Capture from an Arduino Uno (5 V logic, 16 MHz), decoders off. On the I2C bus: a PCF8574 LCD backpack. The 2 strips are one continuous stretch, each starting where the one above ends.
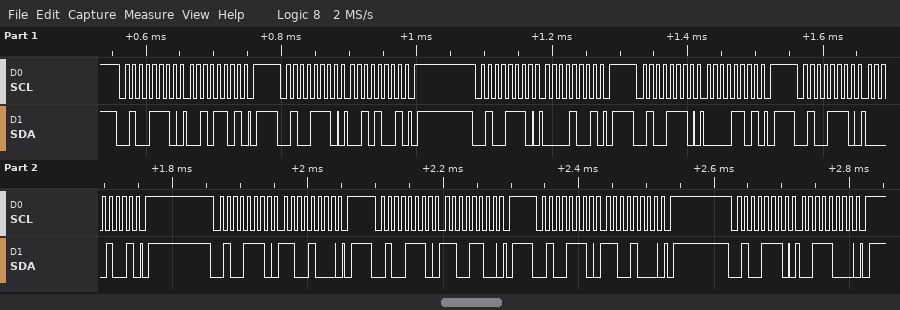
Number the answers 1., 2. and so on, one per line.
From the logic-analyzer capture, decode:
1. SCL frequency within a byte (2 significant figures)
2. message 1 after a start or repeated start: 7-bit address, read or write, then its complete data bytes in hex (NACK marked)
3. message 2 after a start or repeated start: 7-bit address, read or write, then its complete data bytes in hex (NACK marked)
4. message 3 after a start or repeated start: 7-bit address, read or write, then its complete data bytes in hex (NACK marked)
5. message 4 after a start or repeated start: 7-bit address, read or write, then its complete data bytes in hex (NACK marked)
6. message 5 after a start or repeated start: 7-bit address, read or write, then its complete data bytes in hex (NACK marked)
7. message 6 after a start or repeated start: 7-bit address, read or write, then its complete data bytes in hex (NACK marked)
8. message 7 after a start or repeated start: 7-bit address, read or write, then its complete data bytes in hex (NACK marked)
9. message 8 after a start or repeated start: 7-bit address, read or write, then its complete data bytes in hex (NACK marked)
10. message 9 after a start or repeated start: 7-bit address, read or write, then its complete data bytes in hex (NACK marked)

1. 100 kHz
2. 0x27 write: 2D
3. 0x27 write: 29
4. 0x27 write: 09
5. 0x27 write: 0D
6. 0x27 write: 09
7. 0x27 write: C8
8. 0x27 write: CC
9. 0x27 write: C8
10. 0x27 write: 38
